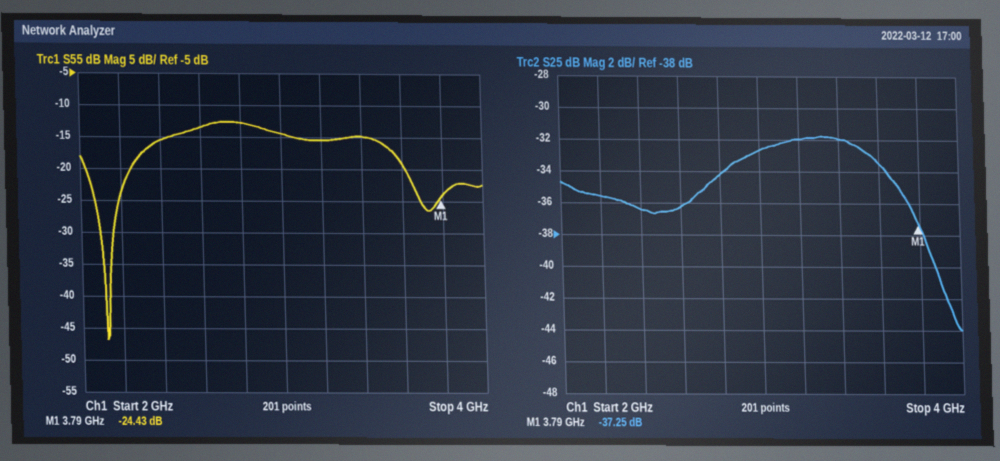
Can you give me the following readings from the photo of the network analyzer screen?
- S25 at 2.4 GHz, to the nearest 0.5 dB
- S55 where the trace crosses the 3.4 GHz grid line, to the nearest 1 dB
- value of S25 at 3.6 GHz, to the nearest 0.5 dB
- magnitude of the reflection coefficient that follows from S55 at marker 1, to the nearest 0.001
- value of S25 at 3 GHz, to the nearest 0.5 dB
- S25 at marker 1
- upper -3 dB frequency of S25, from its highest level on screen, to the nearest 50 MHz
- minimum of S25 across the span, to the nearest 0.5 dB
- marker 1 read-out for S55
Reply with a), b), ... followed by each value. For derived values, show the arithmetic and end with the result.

a) -36.5 dB
b) -15 dB
c) -33.5 dB
d) 10^(-24.43/20) ≈ 0.060
e) -32.5 dB
f) -37.25 dB
g) 3.70 GHz
h) -44.0 dB
i) -24.43 dB
